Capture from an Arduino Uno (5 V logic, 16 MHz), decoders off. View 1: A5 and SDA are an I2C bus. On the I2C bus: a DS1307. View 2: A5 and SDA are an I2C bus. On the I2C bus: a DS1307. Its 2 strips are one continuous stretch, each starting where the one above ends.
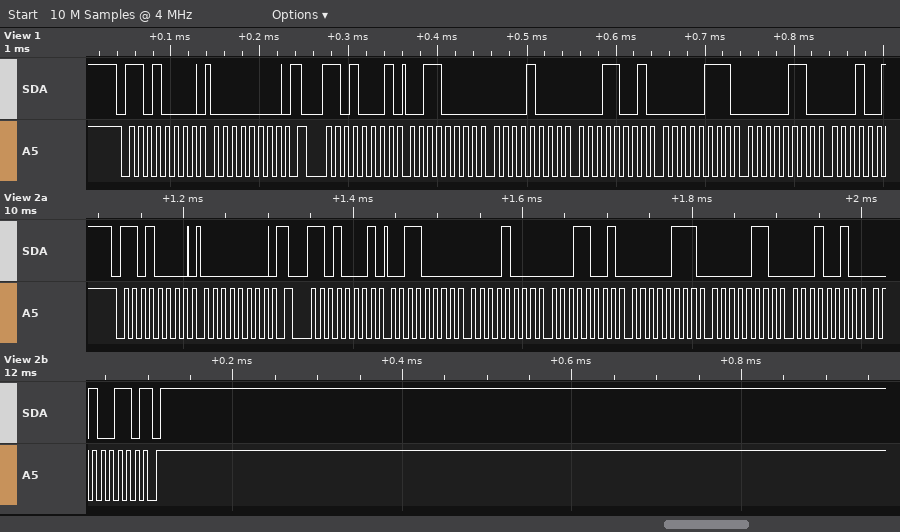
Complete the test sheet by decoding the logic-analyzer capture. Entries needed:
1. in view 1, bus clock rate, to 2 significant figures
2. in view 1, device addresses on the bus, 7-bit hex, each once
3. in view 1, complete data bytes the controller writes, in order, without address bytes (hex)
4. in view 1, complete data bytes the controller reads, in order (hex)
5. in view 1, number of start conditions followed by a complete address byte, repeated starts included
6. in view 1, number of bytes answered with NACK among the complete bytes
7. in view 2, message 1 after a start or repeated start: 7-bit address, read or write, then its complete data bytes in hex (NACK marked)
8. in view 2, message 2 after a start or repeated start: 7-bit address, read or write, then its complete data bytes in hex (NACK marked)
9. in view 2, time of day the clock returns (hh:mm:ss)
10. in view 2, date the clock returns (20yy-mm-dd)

100 kHz
0x68
00
30 08 19 07 06
2
0
0x68 write: 00
0x68 read: 30 08 19 07 06 12 26 NACK
19:08:30
2026-12-06
